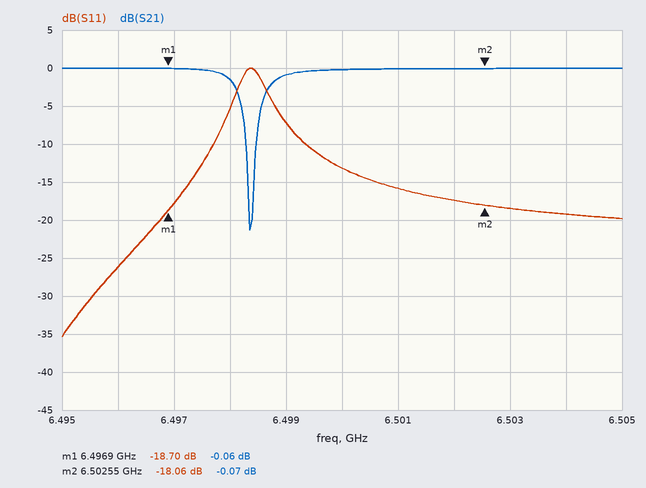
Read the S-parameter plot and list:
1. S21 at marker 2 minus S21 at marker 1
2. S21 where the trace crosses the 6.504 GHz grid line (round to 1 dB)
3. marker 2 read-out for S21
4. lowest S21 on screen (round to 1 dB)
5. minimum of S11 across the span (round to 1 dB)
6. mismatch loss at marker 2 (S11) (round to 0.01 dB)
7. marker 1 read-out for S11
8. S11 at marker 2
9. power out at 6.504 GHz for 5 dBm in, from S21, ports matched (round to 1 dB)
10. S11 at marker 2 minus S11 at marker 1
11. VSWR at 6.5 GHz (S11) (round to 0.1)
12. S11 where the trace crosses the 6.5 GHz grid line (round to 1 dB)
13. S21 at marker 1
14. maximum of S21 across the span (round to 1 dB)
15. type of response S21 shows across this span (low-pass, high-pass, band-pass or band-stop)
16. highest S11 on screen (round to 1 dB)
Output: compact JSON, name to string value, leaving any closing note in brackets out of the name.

{"S21 at marker 2 minus S21 at marker 1": "-0.01 dB", "S21 where the trace crosses the 6.504 GHz grid line": "0 dB", "marker 2 read-out for S21": "-0.07 dB", "lowest S21 on screen": "-21 dB", "minimum of S11 across the span": "-35 dB", "mismatch loss at marker 2 (S11)": "0.07 dB", "marker 1 read-out for S11": "-18.70 dB", "S11 at marker 2": "-18.06 dB", "power out at 6.504 GHz for 5 dBm in, from S21, ports matched": "5 dBm", "S11 at marker 2 minus S11 at marker 1": "0.64 dB", "VSWR at 6.5 GHz (S11)": "1.6", "S11 where the trace crosses the 6.5 GHz grid line": "-13 dB", "S21 at marker 1": "-0.06 dB", "maximum of S21 across the span": "0 dB", "type of response S21 shows across this span": "band-stop", "highest S11 on screen": "0 dB"}
